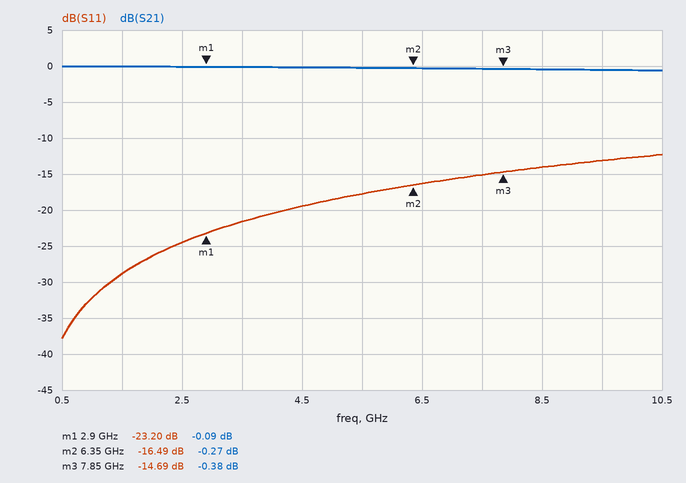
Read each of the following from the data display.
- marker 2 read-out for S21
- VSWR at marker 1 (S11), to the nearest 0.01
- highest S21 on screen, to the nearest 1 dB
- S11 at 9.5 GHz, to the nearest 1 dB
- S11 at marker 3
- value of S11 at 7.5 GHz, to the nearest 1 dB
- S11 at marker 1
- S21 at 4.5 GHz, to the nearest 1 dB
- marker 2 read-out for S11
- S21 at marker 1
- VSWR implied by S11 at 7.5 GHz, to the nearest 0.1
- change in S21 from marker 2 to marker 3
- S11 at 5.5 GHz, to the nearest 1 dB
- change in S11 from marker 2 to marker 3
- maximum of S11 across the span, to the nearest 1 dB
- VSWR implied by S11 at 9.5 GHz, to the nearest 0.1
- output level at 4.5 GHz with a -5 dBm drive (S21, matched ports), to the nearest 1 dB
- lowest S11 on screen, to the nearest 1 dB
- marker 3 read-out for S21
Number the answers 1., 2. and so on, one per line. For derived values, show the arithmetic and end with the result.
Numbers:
1. -0.27 dB
2. (1 + 0.0692)/(1 − 0.0692) ≈ 1.15
3. 0 dB
4. -13 dB
5. -14.69 dB
6. -15 dB
7. -23.20 dB
8. 0 dB
9. -16.49 dB
10. -0.09 dB
11. |Γ| = 10^(-15/20) = 0.1778; VSWR = (1 + 0.1778)/(1 − 0.1778) ≈ 1.4
12. -0.38 − (-0.27) = -0.11 dB
13. -18 dB
14. -14.69 − (-16.49) = 1.80 dB
15. -12 dB
16. |Γ| = 10^(-13/20) = 0.2239; VSWR = (1 + 0.2239)/(1 − 0.2239) ≈ 1.6
17. -5 dBm + (0 dB) = -5 dBm
18. -38 dB
19. -0.38 dB
